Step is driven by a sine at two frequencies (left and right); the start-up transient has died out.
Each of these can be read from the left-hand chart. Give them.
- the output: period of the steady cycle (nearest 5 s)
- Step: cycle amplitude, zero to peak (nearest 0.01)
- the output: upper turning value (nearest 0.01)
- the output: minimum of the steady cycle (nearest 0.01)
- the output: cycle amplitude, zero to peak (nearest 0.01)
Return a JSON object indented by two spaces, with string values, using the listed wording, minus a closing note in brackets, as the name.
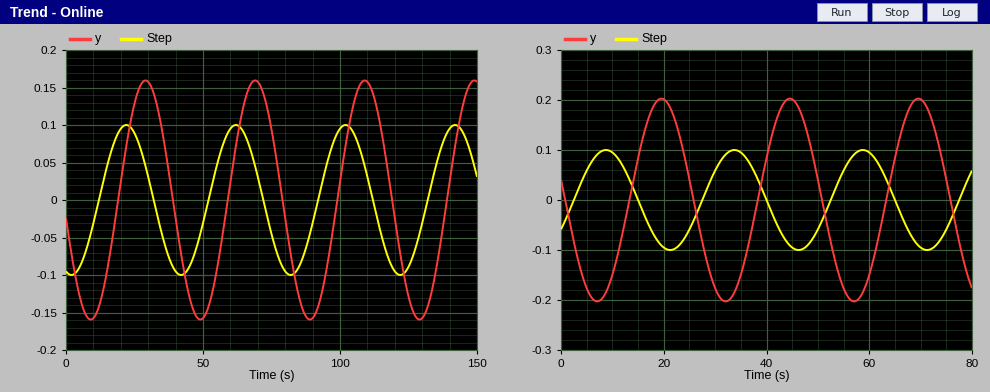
{
  "the output: period of the steady cycle": "40 s",
  "Step: cycle amplitude, zero to peak": "0.10",
  "the output: upper turning value": "0.16",
  "the output: minimum of the steady cycle": "-0.16",
  "the output: cycle amplitude, zero to peak": "0.16"
}
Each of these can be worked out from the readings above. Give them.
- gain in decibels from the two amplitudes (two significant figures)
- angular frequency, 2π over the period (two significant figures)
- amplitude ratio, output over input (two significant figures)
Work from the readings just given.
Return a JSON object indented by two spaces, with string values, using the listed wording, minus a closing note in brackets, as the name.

{
  "gain in decibels from the two amplitudes": "4.1 dB",
  "angular frequency, 2π over the period": "0.16 rad/s",
  "amplitude ratio, output over input": "1.6"
}
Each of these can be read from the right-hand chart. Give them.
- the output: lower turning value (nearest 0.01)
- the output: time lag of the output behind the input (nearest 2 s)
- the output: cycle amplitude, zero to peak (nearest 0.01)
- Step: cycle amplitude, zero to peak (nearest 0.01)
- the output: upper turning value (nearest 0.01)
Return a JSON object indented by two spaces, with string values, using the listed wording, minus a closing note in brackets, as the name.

{
  "the output: lower turning value": "-0.20",
  "the output: time lag of the output behind the input": "10 s",
  "the output: cycle amplitude, zero to peak": "0.20",
  "Step: cycle amplitude, zero to peak": "0.10",
  "the output: upper turning value": "0.20"
}
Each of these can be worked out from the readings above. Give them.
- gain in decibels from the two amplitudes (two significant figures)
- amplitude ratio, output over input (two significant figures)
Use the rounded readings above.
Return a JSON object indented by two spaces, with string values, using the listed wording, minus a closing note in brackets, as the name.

{
  "gain in decibels from the two amplitudes": "6.0 dB",
  "amplitude ratio, output over input": "2.0"
}
